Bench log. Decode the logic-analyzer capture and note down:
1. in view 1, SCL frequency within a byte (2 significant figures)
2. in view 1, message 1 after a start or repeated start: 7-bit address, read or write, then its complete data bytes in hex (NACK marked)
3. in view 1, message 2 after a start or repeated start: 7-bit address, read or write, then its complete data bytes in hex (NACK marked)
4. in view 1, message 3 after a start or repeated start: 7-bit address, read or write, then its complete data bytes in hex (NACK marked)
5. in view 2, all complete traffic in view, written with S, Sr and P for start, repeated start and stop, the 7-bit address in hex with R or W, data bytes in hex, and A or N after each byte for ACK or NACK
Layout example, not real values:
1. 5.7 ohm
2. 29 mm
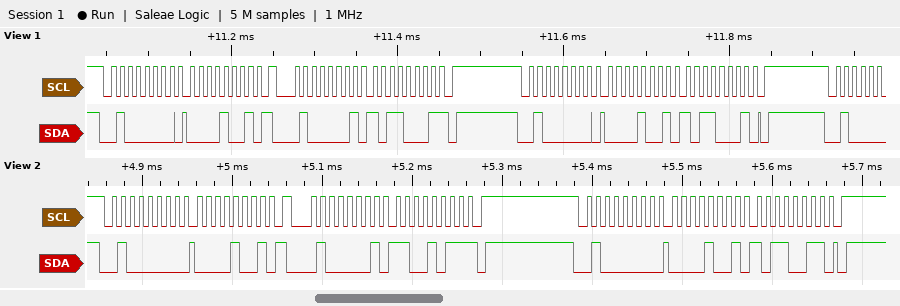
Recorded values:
1. 100 kHz
2. 0x20 write: 09
3. 0x20 read: B1 NACK
4. 0x20 write: 09 B1
5. S 20W A 09 A Sr 20R A CB N P S 20W A 09 A B3 A P
